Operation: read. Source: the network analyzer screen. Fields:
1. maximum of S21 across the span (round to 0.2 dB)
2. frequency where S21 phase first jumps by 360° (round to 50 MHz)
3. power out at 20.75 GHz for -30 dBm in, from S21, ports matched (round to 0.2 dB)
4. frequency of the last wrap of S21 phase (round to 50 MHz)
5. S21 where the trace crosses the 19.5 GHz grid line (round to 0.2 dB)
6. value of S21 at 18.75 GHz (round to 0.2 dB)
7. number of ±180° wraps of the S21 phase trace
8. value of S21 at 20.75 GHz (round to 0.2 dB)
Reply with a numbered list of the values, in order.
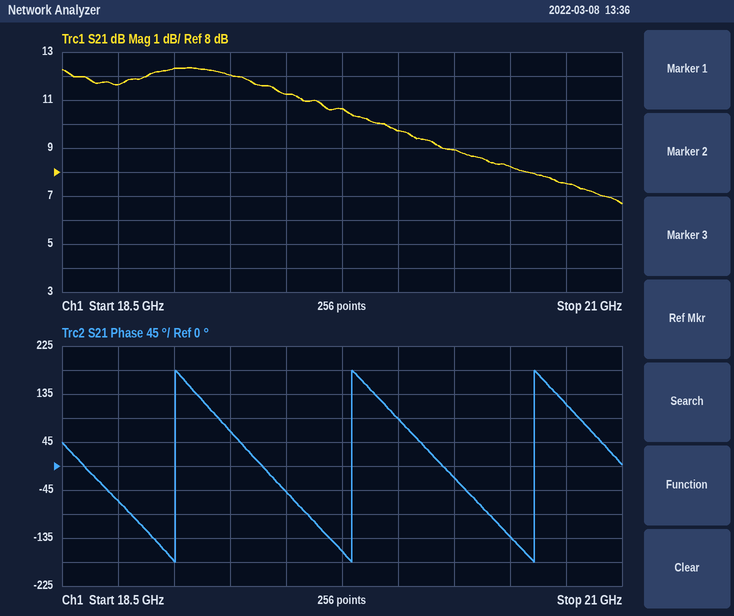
1. 12.4 dB
2. 19.00 GHz
3. -22.4 dBm
4. 20.60 GHz
5. 11.2 dB
6. 11.6 dB
7. 3
8. 7.6 dB
